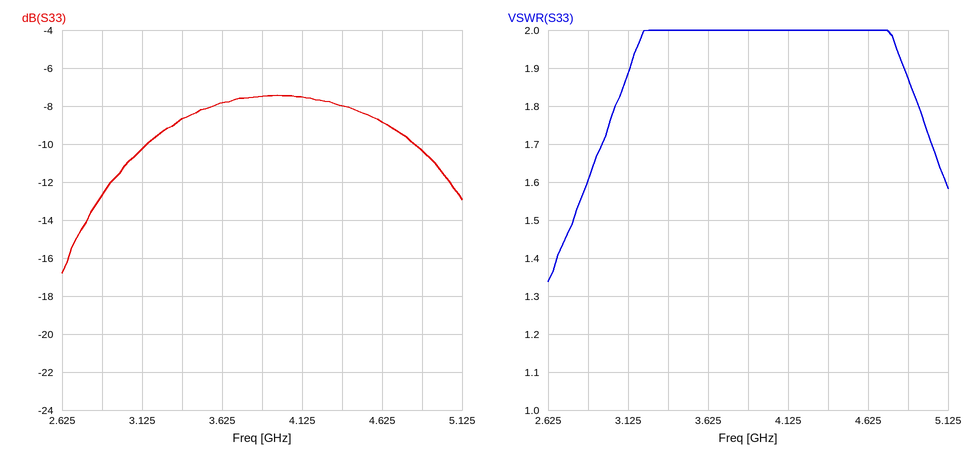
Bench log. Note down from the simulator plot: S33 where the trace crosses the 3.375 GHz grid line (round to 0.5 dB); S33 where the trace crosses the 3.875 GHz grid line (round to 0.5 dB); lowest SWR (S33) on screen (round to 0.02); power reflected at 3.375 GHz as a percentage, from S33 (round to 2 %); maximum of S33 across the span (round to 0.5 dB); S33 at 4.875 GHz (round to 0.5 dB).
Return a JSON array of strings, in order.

["-8.5 dB", "-7.5 dB", "1.34", "14 %", "-7.5 dB", "-10.5 dB"]
